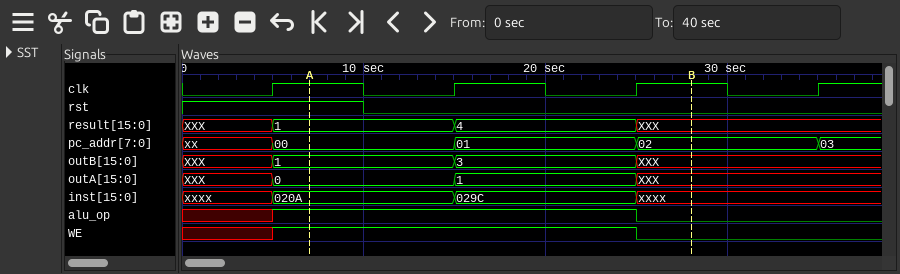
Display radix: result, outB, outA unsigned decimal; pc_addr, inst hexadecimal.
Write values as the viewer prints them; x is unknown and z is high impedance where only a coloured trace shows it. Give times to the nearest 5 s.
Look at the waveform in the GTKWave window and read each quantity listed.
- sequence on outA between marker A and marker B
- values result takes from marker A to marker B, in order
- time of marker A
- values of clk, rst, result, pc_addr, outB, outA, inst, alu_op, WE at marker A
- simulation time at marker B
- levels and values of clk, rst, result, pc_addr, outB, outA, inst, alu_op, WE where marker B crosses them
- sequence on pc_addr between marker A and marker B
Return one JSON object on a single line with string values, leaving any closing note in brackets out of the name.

{"sequence on outA between marker A and marker B": "0, 1, XXX", "values result takes from marker A to marker B, in order": "1, 4, XXX", "time of marker A": "5 s", "values of clk, rst, result, pc_addr, outB, outA, inst, alu_op, WE at marker A": "clk=1, rst=1, result=1, pc_addr=00, outB=1, outA=0, inst=020A, alu_op=1, WE=1", "simulation time at marker B": "30 s", "levels and values of clk, rst, result, pc_addr, outB, outA, inst, alu_op, WE where marker B crosses them": "clk=1, rst=0, result=XXX, pc_addr=02, outB=XXX, outA=XXX, inst=xxxx, alu_op=0, WE=0", "sequence on pc_addr between marker A and marker B": "00, 01, 02"}
